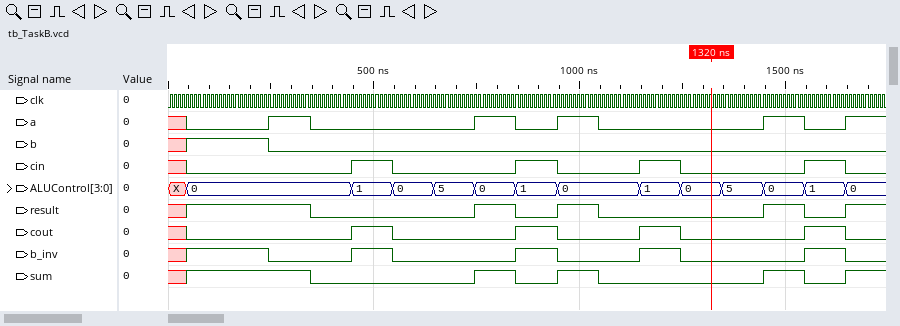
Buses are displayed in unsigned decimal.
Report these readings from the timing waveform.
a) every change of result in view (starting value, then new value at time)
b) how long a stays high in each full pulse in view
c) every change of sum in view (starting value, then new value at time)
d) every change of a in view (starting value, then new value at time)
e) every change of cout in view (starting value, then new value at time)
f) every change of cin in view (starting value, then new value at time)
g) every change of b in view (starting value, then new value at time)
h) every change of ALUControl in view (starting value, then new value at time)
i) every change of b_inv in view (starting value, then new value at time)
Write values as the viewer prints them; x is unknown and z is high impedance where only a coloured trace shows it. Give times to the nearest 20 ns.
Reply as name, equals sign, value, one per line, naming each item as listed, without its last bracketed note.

every change of result in view = x, 1 at 40 ns, 0 at 340 ns, 1 at 740 ns, 0 at 840 ns, 1 at 940 ns, 0 at 1040 ns, 1 at 1440 ns, 0 at 1540 ns, 1 at 1640 ns
how long a stays high in each full pulse in view = 100 ns, 100 ns, 100 ns, 100 ns
every change of sum in view = x, 1 at 40 ns, 0 at 340 ns, 1 at 740 ns, 0 at 840 ns, 1 at 940 ns, 0 at 1040 ns, 1 at 1440 ns, 0 at 1540 ns, 1 at 1640 ns
every change of a in view = x, 0 at 40 ns, 1 at 240 ns, 0 at 340 ns, 1 at 740 ns, 0 at 840 ns, 1 at 940 ns, 0 at 1040 ns, 1 at 1440 ns, 0 at 1540 ns, 1 at 1640 ns
every change of cout in view = x, 0 at 40 ns, 1 at 440 ns, 0 at 540 ns, 1 at 840 ns, 0 at 940 ns, 1 at 1140 ns, 0 at 1240 ns, 1 at 1540 ns, 0 at 1640 ns
every change of cin in view = x, 0 at 40 ns, 1 at 440 ns, 0 at 540 ns, 1 at 840 ns, 0 at 940 ns, 1 at 1140 ns, 0 at 1240 ns, 1 at 1540 ns, 0 at 1640 ns
every change of b in view = x, 1 at 40 ns, 0 at 240 ns
every change of ALUControl in view = X, 0 at 40 ns, 1 at 440 ns, 0 at 540 ns, 5 at 640 ns, 0 at 740 ns, 1 at 840 ns, 0 at 940 ns, 1 at 1140 ns, 0 at 1240 ns, 5 at 1340 ns, 0 at 1440 ns, 1 at 1540 ns, 0 at 1640 ns
every change of b_inv in view = x, 1 at 40 ns, 0 at 240 ns, 1 at 440 ns, 0 at 540 ns, 1 at 840 ns, 0 at 940 ns, 1 at 1140 ns, 0 at 1240 ns, 1 at 1540 ns, 0 at 1640 ns
